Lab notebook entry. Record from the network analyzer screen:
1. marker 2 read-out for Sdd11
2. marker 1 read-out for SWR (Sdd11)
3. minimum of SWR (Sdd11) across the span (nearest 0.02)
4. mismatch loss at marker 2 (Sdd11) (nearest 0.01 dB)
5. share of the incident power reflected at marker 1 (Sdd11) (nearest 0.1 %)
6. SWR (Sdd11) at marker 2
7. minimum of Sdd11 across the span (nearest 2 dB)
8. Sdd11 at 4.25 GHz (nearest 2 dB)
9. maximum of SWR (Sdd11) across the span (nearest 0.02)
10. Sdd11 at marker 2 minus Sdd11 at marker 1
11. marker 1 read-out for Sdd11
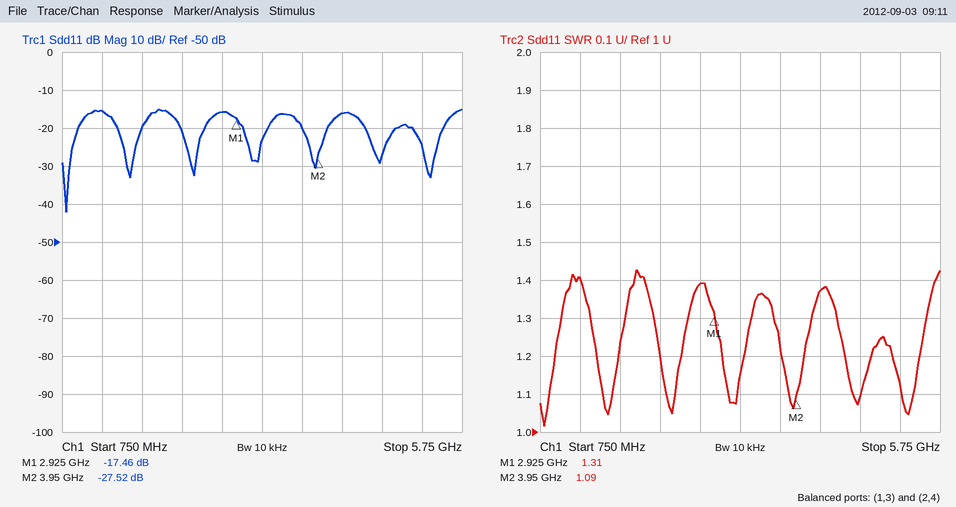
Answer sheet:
-27.52 dB
1.31
1.02
0.01 dB
1.8 %
1.09
-42 dB
-16 dB
1.42
-10.06 dB
-17.46 dB
